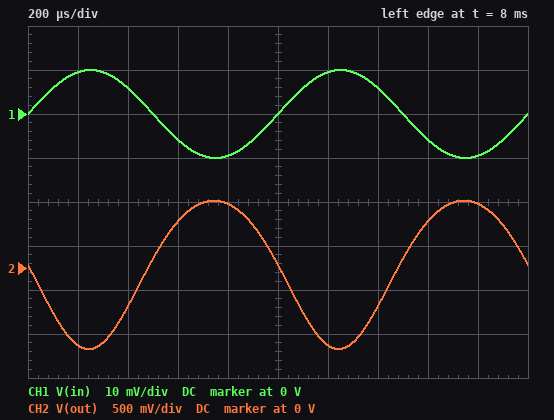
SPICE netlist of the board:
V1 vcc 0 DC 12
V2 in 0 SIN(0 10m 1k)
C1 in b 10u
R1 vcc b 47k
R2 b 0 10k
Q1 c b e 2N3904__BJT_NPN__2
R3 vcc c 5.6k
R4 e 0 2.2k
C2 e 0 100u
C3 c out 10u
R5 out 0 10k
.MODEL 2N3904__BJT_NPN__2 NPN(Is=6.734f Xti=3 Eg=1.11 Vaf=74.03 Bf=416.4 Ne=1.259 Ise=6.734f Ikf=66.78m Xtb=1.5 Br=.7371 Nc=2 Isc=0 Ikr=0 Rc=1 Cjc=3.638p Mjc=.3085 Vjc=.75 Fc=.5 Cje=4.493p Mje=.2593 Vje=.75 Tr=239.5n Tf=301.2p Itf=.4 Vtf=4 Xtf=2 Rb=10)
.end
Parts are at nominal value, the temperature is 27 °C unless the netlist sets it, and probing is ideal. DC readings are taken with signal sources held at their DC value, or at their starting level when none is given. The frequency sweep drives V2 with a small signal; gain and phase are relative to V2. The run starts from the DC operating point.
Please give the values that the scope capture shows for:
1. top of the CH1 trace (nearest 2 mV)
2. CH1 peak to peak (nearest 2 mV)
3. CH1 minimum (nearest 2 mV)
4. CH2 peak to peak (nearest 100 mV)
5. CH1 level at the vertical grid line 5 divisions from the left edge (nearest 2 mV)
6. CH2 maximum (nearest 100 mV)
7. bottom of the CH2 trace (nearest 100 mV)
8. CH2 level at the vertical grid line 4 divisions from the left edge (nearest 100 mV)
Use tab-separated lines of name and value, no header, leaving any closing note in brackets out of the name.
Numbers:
top of the CH1 trace	10 mV
CH1 peak to peak	20 mV
CH1 minimum	-10 mV
CH2 peak to peak	1.7 V
CH1 level at the vertical grid line 5 divisions from the left edge	0 V
CH2 maximum	800 mV
bottom of the CH2 trace	-900 mV
CH2 level at the vertical grid line 4 divisions from the left edge	700 mV
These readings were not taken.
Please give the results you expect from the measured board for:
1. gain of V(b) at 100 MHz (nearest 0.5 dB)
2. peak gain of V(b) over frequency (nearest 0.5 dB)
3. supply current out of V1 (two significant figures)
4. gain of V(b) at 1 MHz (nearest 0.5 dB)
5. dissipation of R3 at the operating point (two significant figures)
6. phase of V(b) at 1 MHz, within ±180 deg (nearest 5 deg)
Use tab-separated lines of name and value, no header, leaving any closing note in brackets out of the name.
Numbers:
gain of V(b) at 100 MHz	0 dB
peak gain of V(b) over frequency	0 dB
supply current out of V1	850 µA
gain of V(b) at 1 MHz	0 dB
dissipation of R3 at the operating point	2.3 mW
phase of V(b) at 1 MHz, within ±180 deg	0 deg
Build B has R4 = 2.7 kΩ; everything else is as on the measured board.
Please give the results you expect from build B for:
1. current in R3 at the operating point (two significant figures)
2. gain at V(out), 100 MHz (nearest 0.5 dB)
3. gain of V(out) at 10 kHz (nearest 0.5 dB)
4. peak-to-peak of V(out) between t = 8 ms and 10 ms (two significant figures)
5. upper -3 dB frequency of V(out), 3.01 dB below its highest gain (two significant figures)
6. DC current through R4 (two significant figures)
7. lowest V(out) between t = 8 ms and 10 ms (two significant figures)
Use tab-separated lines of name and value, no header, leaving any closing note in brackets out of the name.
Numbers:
current in R3 at the operating point	520 µA
gain at V(out), 100 MHz	23.5 dB
gain of V(out) at 10 kHz	37.0 dB
peak-to-peak of V(out) between t = 8 ms and 10 ms	1.4 V
upper -3 dB frequency of V(out), 3.01 dB below its highest gain	21 MHz
DC current through R4	530 µA
lowest V(out) between t = 8 ms and 10 ms	-770 mV
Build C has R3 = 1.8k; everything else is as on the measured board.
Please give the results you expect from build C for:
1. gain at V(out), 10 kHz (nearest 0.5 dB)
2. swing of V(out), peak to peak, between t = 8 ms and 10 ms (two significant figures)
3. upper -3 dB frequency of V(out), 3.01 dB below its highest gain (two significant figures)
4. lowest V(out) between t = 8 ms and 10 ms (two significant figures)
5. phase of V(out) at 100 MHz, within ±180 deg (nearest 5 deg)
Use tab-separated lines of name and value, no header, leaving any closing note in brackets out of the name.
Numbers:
gain at V(out), 10 kHz	31.5 dB
swing of V(out), peak to peak, between t = 8 ms and 10 ms	730 mV
upper -3 dB frequency of V(out), 3.01 dB below its highest gain	50 MHz
lowest V(out) between t = 8 ms and 10 ms	-400 mV
phase of V(out) at 100 MHz, within ±180 deg	110 deg
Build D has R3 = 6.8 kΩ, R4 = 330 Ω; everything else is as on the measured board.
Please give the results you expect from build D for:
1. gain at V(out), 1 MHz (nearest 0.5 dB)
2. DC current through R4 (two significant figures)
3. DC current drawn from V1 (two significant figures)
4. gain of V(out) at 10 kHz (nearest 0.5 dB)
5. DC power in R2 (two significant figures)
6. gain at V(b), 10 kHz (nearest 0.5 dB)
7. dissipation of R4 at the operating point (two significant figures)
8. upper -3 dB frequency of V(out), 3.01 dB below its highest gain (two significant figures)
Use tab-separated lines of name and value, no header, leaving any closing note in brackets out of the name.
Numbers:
gain at V(out), 1 MHz	15.5 dB
DC current through R4	1.8 mA
DC current drawn from V1	1.9 mA
gain of V(out) at 10 kHz	17.5 dB
DC power in R2	160 µW
gain at V(b), 10 kHz	0 dB
dissipation of R4 at the operating point	1.0 mW
upper -3 dB frequency of V(out), 3.01 dB below its highest gain	1.3 MHz
